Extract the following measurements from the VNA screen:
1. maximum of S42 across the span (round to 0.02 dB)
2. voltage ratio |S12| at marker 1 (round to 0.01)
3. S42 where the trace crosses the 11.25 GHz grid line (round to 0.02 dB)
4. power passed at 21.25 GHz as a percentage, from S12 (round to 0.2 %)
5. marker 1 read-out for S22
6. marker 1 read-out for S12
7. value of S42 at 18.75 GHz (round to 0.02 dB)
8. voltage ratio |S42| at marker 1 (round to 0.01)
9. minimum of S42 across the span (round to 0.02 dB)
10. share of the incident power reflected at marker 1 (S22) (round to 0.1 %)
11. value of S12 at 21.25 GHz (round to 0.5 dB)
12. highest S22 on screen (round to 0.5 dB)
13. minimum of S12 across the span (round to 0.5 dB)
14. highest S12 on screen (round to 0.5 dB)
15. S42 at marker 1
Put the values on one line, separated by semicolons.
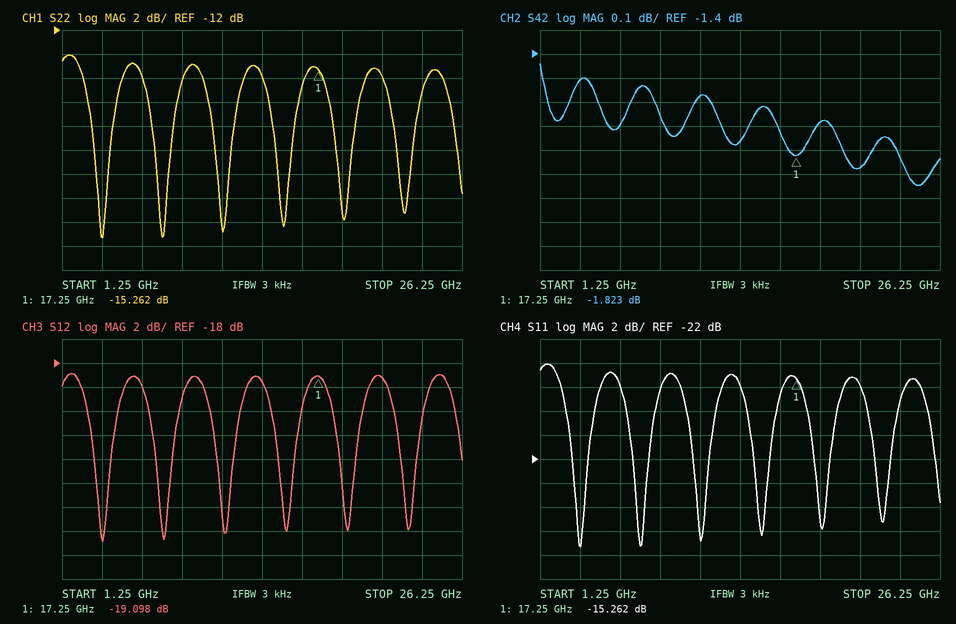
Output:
-1.44 dB; 0.11; -1.58 dB; 1.2 %; -15.262 dB; -19.098 dB; -1.68 dB; 0.81; -1.94 dB; 3.0 %; -19.0 dB; -14.0 dB; -33.0 dB; -19.0 dB; -1.823 dB
